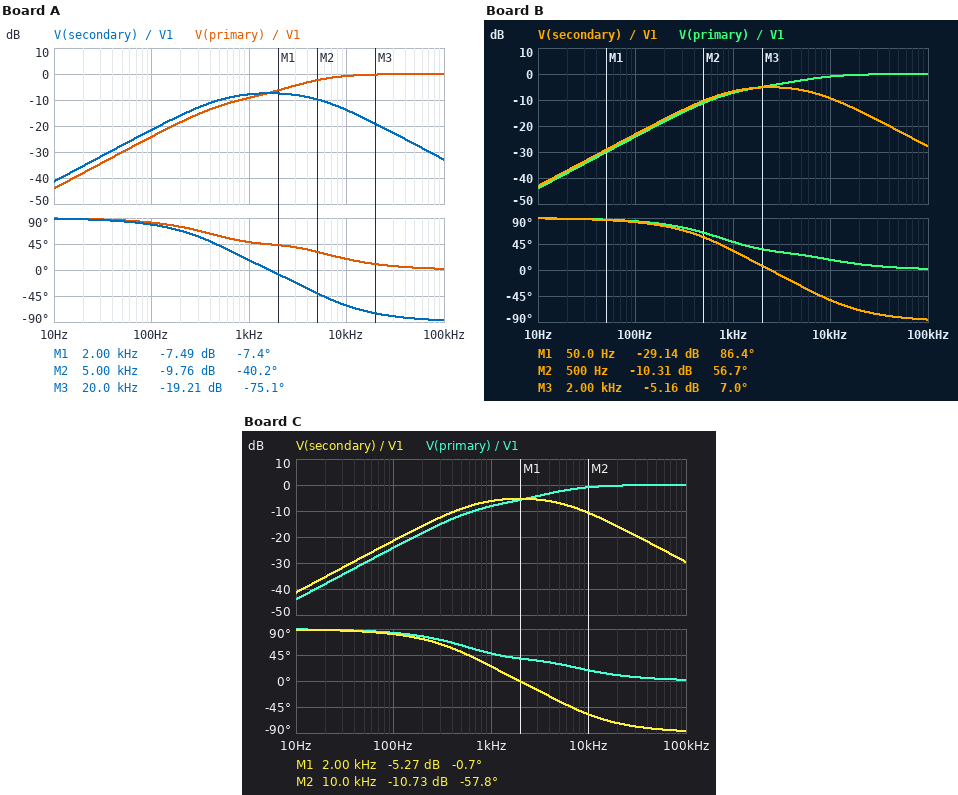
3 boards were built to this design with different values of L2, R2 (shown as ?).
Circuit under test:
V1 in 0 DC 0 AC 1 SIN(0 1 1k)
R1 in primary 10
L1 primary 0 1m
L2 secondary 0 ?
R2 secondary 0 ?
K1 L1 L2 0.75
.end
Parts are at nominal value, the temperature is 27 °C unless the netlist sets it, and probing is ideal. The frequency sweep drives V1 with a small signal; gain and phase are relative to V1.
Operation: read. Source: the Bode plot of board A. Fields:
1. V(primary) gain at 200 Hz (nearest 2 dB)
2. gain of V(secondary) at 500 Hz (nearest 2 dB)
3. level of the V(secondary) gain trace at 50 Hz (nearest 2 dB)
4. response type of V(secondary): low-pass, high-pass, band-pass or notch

-18 dB
-10 dB
-28 dB
band-pass
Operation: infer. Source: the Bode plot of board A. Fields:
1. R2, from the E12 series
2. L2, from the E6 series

15 Ω
3.3 mH
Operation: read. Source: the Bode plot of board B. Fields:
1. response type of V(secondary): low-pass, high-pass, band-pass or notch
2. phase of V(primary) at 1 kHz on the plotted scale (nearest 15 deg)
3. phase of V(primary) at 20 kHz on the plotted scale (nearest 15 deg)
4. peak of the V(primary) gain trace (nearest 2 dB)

band-pass
45 deg
15 deg
0 dB
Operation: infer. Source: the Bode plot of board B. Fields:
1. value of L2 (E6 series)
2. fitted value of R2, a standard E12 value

2.2 mH
22 Ω
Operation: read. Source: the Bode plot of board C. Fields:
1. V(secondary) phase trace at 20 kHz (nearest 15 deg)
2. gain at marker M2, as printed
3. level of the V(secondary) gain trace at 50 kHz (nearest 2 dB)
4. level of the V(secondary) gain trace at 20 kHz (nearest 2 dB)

-75 deg
-10.73 dB
-24 dB
-16 dB
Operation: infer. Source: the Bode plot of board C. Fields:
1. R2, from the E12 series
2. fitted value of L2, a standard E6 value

22 Ω
3.3 mH
